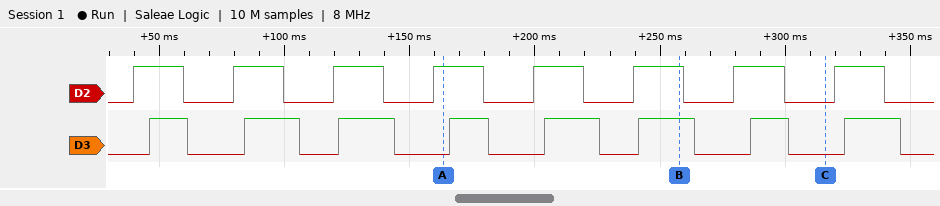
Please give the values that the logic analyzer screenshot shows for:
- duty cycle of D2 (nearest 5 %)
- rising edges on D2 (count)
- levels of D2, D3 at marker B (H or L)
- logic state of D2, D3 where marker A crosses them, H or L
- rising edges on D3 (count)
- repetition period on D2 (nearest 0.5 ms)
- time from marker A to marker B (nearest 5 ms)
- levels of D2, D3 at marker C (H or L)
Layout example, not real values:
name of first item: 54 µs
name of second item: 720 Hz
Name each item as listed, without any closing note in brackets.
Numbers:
duty cycle of D2: 50 %
rising edges on D2: 8
levels of D2, D3 at marker B: D2=H, D3=H
logic state of D2, D3 where marker A crosses them, H or L: D2=H, D3=L
rising edges on D3: 8
repetition period on D2: 40 ms
time from marker A to marker B: 95 ms
levels of D2, D3 at marker C: D2=L, D3=L
